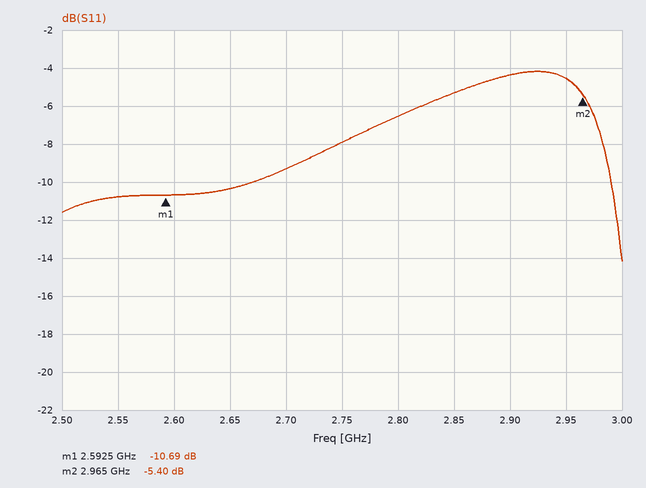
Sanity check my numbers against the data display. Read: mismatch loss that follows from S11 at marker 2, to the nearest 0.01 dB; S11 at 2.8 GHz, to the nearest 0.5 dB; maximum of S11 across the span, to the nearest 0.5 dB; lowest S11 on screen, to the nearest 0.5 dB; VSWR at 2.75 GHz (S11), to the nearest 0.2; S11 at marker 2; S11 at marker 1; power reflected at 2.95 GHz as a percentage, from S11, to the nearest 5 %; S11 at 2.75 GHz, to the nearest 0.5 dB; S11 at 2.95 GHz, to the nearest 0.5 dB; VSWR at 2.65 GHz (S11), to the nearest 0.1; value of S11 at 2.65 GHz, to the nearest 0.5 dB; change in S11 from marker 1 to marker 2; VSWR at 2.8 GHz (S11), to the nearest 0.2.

1.48 dB
-6.5 dB
-4.0 dB
-14.0 dB
2.4
-5.40 dB
-10.69 dB
35 %
-8.0 dB
-4.5 dB
1.9
-10.5 dB
5.29 dB
2.8
